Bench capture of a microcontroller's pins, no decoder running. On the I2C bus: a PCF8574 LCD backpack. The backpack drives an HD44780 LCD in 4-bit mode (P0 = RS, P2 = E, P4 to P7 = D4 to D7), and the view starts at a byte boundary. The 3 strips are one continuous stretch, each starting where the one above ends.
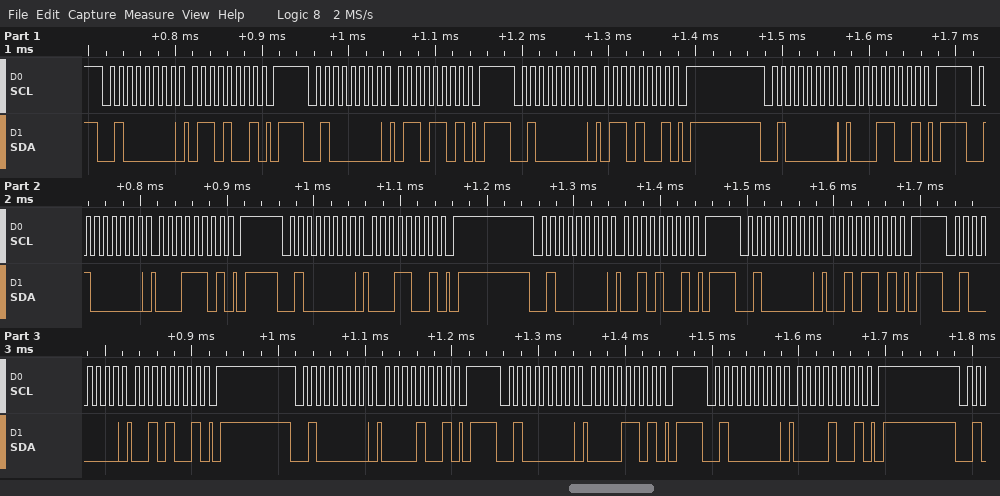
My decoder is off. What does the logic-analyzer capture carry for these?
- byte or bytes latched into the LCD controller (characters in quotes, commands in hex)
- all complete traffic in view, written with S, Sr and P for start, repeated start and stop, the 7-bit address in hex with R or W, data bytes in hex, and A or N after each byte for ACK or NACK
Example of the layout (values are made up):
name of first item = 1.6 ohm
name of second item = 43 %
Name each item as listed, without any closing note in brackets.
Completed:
byte or bytes latched into the LCD controller = 'a' ' '
all complete traffic in view, written with S, Sr and P for start, repeated start and stop, the 7-bit address in hex with R or W, data bytes in hex, and A or N after each byte for ACK or NACK = S 20W A 69 A P S 20W A 6D A P S 20W A 69 A P S 20W A 19 A P S 20W A 1D A P S 20W A 19 A P S 20W A 29 A P S 20W A 2D A P S 20W A 29 A P S 20W A 09 A P S 20W A 0D A P S 20W A 09 A P
